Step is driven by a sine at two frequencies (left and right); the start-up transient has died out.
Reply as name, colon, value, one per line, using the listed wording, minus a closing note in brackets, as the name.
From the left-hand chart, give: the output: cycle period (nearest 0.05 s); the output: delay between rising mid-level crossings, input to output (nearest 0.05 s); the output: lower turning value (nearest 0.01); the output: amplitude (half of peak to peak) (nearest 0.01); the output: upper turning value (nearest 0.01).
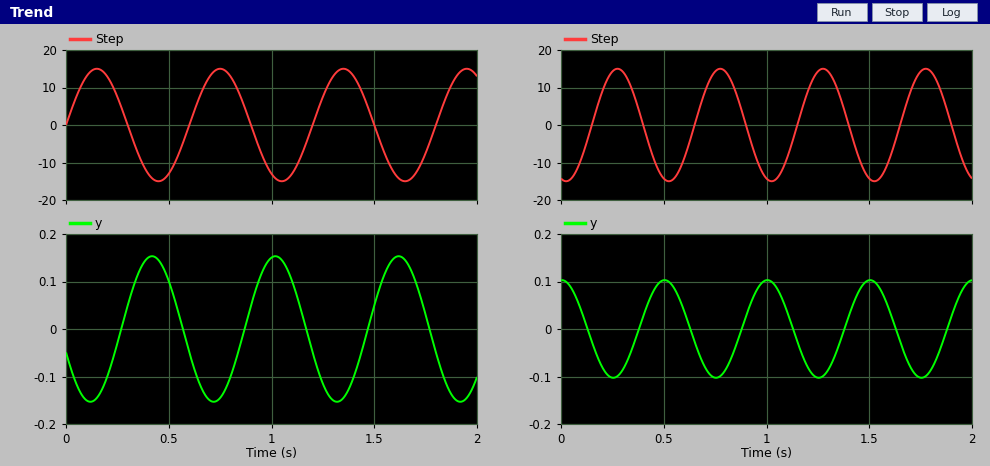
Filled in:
the output: cycle period: 0.60 s
the output: delay between rising mid-level crossings, input to output: 0.25 s
the output: lower turning value: -0.15
the output: amplitude (half of peak to peak): 0.15
the output: upper turning value: 0.15
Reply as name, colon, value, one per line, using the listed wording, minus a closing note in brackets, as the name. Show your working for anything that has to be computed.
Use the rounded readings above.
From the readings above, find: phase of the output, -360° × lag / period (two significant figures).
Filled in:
phase of the output, -360° × lag / period: -360 × 0.25 / 0.6 = -150°
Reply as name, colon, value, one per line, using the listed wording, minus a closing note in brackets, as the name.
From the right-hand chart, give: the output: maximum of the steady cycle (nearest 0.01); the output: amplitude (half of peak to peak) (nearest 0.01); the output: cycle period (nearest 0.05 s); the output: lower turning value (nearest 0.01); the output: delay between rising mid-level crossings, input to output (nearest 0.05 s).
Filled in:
the output: maximum of the steady cycle: 0.10
the output: amplitude (half of peak to peak): 0.10
the output: cycle period: 0.50 s
the output: lower turning value: -0.10
the output: delay between rising mid-level crossings, input to output: 0.25 s
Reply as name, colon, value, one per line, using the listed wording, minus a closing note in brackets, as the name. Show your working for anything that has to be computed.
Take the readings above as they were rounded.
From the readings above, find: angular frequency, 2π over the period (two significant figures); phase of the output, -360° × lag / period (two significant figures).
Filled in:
angular frequency, 2π over the period: 2π / 0.5 = 13 rad/s
phase of the output, -360° × lag / period: -360 × 0.25 / 0.5 = -180°
